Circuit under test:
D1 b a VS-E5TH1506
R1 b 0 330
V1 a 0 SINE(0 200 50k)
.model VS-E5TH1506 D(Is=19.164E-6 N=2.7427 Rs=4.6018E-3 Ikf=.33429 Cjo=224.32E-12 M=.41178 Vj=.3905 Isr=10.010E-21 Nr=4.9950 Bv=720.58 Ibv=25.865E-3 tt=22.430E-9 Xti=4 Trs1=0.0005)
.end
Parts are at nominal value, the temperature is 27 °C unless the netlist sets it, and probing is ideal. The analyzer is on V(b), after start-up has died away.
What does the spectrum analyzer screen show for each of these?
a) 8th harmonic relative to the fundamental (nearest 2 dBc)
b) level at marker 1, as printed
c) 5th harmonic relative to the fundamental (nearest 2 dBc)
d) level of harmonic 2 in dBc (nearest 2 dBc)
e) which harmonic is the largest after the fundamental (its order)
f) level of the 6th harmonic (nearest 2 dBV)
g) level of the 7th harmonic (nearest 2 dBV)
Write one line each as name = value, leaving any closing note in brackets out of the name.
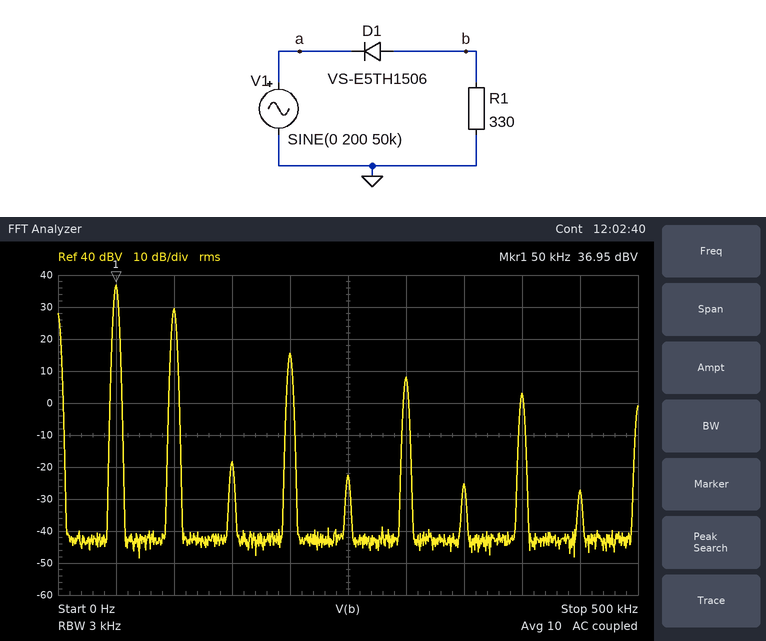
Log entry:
8th harmonic relative to the fundamental = -34 dBc
level at marker 1, as printed = 36.95 dBV
5th harmonic relative to the fundamental = -60 dBc
level of harmonic 2 in dBc = -8 dBc
which harmonic is the largest after the fundamental = 2
level of the 6th harmonic = 8 dBV
level of the 7th harmonic = -26 dBV
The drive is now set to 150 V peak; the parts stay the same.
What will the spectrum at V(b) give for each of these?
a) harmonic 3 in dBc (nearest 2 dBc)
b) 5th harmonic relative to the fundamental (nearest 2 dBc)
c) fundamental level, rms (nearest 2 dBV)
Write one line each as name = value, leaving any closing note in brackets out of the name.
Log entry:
harmonic 3 in dBc = -54 dBc
5th harmonic relative to the fundamental = -58 dBc
fundamental level, rms = 34 dBV
